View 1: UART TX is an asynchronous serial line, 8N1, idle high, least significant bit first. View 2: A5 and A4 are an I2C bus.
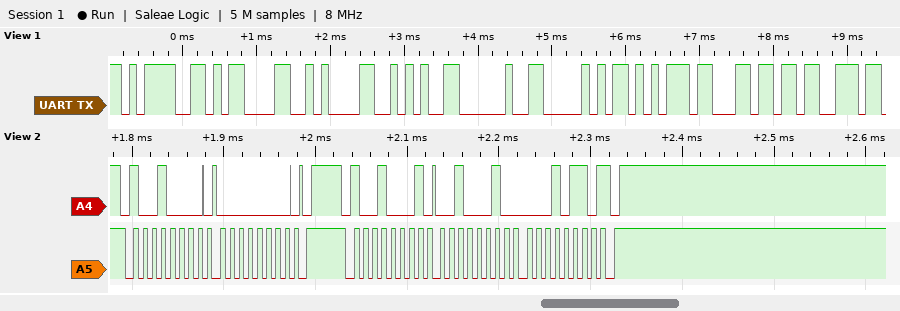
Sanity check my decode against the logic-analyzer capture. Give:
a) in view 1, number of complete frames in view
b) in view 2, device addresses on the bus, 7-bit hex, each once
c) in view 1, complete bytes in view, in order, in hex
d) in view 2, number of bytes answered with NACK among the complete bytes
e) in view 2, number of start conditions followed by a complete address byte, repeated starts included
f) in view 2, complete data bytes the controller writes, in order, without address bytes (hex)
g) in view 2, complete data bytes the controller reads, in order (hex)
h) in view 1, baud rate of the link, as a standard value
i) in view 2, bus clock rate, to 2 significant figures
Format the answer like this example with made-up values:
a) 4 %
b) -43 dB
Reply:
a) 9
b) 0x48
c) 3D 0D 0A 2A 20 50 75 6C 73
d) 1
e) 2
f) 00
g) 22 16
h) 9600 baud
i) 100 kHz
